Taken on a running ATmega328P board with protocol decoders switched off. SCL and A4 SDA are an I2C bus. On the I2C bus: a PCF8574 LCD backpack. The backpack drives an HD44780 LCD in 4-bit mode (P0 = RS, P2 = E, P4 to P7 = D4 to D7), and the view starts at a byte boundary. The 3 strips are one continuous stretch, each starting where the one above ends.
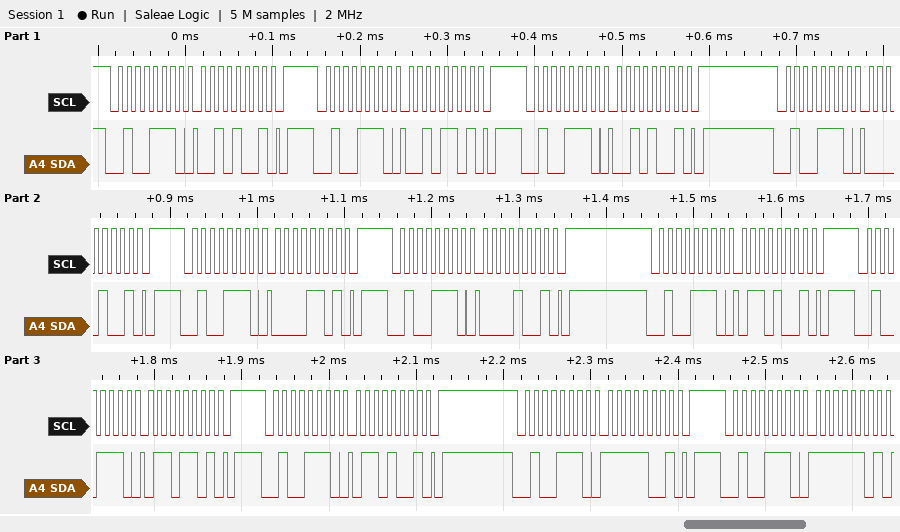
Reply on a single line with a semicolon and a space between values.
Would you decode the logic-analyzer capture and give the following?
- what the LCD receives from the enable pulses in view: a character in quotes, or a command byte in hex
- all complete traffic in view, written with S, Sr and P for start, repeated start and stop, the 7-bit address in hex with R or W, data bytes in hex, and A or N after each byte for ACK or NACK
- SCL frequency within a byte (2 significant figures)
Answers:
' '; S 27W A 29 A P S 27W A 2D A P S 27W A 29 A P S 27W A 09 A P S 27W A 0D A P S 27W A 09 A P S 27W A 69 A P S 27W A 6D A P S 27W A 69 A P S 27W A F9 A P S 27W A FD A; 100 kHz
